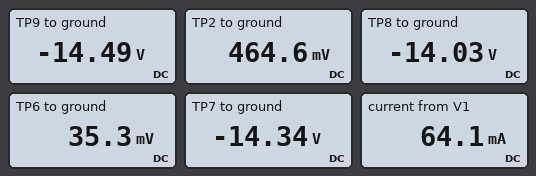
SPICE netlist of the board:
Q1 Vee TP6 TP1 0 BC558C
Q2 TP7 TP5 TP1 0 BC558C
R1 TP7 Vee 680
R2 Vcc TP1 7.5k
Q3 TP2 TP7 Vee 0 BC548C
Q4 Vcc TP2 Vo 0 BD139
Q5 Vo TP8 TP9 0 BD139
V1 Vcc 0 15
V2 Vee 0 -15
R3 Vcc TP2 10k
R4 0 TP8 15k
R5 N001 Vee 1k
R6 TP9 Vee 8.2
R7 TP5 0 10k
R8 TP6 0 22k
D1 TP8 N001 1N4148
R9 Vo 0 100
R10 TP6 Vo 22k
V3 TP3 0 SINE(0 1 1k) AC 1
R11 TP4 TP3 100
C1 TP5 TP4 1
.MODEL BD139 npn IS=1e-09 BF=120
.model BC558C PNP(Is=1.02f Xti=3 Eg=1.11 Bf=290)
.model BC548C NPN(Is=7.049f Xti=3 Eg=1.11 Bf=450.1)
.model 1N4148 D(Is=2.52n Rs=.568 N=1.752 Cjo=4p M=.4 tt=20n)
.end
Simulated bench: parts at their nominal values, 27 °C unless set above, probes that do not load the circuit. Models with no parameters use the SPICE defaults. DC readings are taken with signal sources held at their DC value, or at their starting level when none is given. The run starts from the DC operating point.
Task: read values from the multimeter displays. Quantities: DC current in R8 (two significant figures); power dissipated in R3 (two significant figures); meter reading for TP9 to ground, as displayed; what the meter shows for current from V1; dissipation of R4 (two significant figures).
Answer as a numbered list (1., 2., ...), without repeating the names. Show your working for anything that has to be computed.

1. (35.3 mV) / 22 kΩ = 1.6 µA
2. (15 V - 464.6 mV)^2 / 10 kΩ = 21 mW
3. -14.49 V
4. 64.1 mA
5. (0 V - (-14.03 V))^2 / 15 kΩ = 13 mW
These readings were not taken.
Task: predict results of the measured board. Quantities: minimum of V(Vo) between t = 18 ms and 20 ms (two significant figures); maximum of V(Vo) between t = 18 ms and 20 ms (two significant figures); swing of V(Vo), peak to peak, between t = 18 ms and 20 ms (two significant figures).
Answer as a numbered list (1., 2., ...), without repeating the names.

1. -2.0 V
2. 2.0 V
3. 4.0 V
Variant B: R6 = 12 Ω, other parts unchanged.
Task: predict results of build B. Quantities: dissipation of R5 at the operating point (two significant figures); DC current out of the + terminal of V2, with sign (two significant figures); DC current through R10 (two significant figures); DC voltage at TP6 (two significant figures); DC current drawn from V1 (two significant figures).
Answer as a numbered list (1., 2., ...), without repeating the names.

1. 260 µW
2. -54 mA
3. 1.5 µA
4. 36 mV
5. 53 mA
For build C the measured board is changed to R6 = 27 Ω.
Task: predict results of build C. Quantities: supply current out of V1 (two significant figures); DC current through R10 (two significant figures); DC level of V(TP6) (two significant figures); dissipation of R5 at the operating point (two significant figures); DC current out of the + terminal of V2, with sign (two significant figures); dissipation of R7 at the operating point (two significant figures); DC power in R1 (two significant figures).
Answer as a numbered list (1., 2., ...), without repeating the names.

1. 32 mA
2. 1.5 µA
3. 36 mV
4. 450 µW
5. -33 mA
6. 120 nW
7. 660 µW
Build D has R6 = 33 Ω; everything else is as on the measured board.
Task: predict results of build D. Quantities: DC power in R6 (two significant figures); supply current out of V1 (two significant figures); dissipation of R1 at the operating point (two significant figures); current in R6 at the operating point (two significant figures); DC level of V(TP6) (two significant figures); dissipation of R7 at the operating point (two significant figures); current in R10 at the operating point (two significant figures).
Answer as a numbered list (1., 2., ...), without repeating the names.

1. 21 mW
2. 28 mA
3. 660 µW
4. 25 mA
5. 36 mV
6. 120 nW
7. 1.5 µA
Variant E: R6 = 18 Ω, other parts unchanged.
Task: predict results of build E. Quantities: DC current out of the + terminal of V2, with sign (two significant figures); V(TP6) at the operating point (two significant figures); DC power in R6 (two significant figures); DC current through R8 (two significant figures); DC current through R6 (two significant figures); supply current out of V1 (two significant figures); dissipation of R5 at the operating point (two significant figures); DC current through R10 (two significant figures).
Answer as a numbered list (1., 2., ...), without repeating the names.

1. -43 mA
2. 36 mV
3. 28 mW
4. 1.6 µA
5. 39 mA
6. 42 mA
7. 360 µW
8. 1.5 µA
